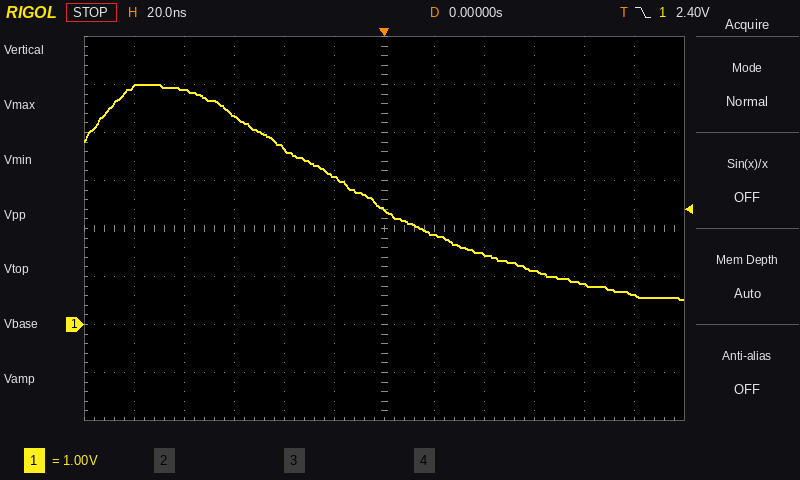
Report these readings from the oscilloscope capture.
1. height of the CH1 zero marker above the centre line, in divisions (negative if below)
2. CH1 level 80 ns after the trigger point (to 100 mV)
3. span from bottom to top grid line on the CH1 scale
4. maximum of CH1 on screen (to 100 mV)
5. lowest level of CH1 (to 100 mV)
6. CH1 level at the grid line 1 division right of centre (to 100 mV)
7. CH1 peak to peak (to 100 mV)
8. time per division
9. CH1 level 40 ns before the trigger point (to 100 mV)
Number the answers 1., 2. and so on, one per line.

1. -2.0 div
2. 800 mV
3. 8 V
4. 5.0 V
5. 500 mV
6. 1.9 V
7. 4.5 V
8. 20 ns
9. 3.7 V
